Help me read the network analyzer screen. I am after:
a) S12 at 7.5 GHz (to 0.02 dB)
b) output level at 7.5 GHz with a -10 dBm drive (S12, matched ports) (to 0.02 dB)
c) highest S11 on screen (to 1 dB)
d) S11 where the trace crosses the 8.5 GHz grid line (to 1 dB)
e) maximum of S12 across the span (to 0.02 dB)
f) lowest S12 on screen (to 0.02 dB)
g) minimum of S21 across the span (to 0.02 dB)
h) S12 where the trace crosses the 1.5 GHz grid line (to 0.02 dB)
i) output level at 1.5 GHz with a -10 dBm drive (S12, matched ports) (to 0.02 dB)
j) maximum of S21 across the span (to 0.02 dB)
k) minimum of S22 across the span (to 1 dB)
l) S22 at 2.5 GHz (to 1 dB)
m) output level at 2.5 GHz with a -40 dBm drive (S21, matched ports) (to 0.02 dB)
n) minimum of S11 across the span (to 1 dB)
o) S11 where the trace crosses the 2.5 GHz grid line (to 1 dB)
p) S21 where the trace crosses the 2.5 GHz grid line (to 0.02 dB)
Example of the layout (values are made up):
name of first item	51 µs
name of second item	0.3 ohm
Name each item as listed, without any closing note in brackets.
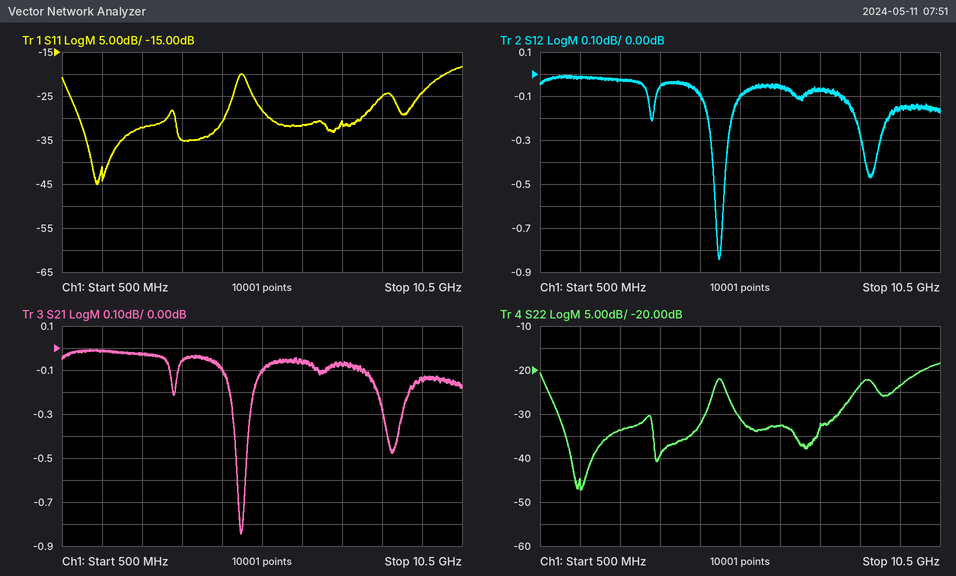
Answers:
S12 at 7.5 GHz	-0.08 dB
output level at 7.5 GHz with a -10 dBm drive (S12, matched ports)	-10.08 dBm
highest S11 on screen	-18 dB
S11 where the trace crosses the 8.5 GHz grid line	-25 dB
maximum of S12 across the span	0.00 dB
lowest S12 on screen	-0.84 dB
minimum of S21 across the span	-0.84 dB
S12 where the trace crosses the 1.5 GHz grid line	-0.02 dB
output level at 1.5 GHz with a -10 dBm drive (S12, matched ports)	-10.02 dBm
maximum of S21 across the span	0.00 dB
minimum of S22 across the span	-47 dB
S22 at 2.5 GHz	-34 dB
output level at 2.5 GHz with a -40 dBm drive (S21, matched ports)	-40.02 dBm
minimum of S11 across the span	-45 dB
S11 where the trace crosses the 2.5 GHz grid line	-32 dB
S21 where the trace crosses the 2.5 GHz grid line	-0.02 dB
